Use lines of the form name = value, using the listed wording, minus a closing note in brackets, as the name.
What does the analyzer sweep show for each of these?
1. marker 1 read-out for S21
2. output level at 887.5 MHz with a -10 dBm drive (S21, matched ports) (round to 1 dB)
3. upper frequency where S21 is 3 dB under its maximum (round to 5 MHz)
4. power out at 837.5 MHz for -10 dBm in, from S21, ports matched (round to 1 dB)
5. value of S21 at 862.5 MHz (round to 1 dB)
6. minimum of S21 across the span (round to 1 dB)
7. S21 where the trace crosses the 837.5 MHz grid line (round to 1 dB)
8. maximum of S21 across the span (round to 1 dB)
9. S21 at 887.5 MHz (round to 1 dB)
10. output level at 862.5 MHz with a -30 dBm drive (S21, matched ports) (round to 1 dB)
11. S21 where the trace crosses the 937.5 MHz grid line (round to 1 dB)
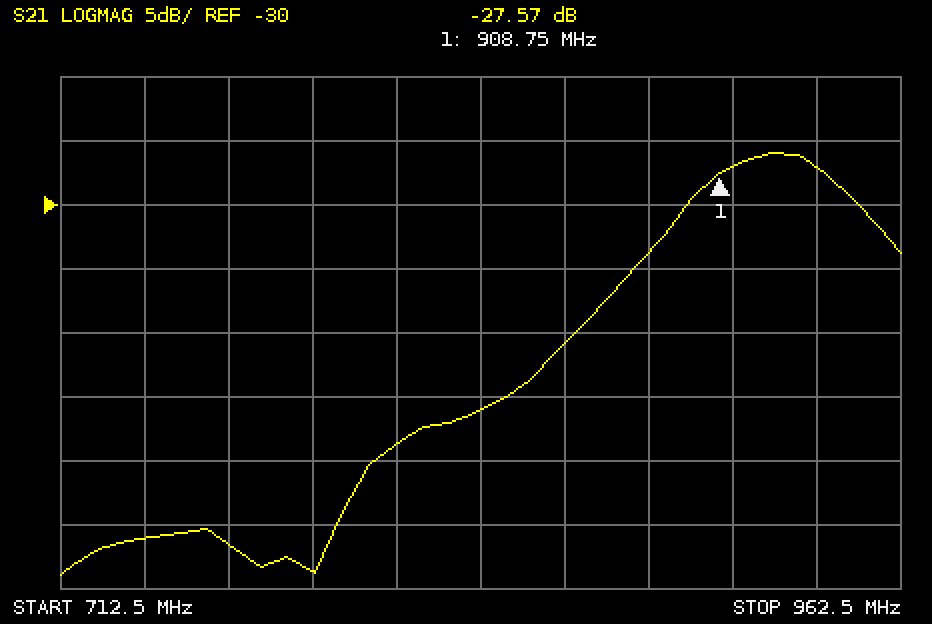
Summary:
marker 1 read-out for S21 = -27.57 dB
output level at 887.5 MHz with a -10 dBm drive (S21, matched ports) = -44 dBm
upper frequency where S21 is 3 dB under its maximum = 945 MHz
power out at 837.5 MHz for -10 dBm in, from S21, ports matched = -56 dBm
value of S21 at 862.5 MHz = -41 dB
minimum of S21 across the span = -59 dB
S21 where the trace crosses the 837.5 MHz grid line = -46 dB
maximum of S21 across the span = -26 dB
S21 at 887.5 MHz = -34 dB
output level at 862.5 MHz with a -30 dBm drive (S21, matched ports) = -71 dBm
S21 where the trace crosses the 937.5 MHz grid line = -27 dB
